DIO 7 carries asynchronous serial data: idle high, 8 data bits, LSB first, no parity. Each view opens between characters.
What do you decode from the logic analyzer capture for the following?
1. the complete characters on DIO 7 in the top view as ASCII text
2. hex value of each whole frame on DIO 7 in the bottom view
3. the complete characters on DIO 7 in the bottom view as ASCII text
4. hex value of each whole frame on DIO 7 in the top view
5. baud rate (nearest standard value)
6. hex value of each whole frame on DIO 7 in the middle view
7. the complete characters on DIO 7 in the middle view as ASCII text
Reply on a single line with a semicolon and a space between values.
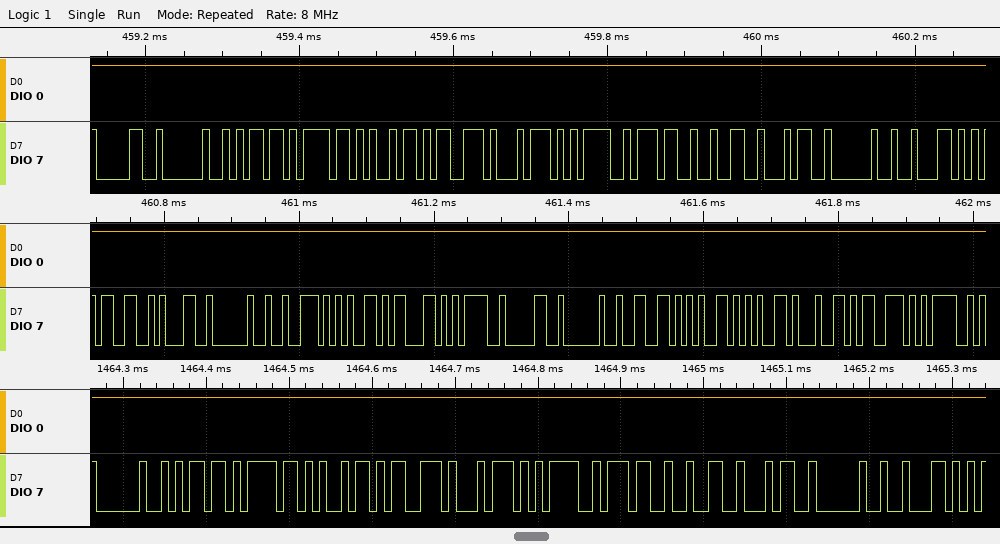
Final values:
"0 moist=724 b"; 20, 6D, 6F, 69, 73, 74, 3D, 37, 32, 34, 20, 62; " moist=724 b"; 30, 20, 6D, 6F, 69, 73, 74, 3D, 37, 32, 34, 20, 62; 115200 baud; 33, 31, 20, 72, 65, 63, 3D, 30, 20, 66, 65, 65, 64, 73, 3D; "31 rec=0 feeds="
